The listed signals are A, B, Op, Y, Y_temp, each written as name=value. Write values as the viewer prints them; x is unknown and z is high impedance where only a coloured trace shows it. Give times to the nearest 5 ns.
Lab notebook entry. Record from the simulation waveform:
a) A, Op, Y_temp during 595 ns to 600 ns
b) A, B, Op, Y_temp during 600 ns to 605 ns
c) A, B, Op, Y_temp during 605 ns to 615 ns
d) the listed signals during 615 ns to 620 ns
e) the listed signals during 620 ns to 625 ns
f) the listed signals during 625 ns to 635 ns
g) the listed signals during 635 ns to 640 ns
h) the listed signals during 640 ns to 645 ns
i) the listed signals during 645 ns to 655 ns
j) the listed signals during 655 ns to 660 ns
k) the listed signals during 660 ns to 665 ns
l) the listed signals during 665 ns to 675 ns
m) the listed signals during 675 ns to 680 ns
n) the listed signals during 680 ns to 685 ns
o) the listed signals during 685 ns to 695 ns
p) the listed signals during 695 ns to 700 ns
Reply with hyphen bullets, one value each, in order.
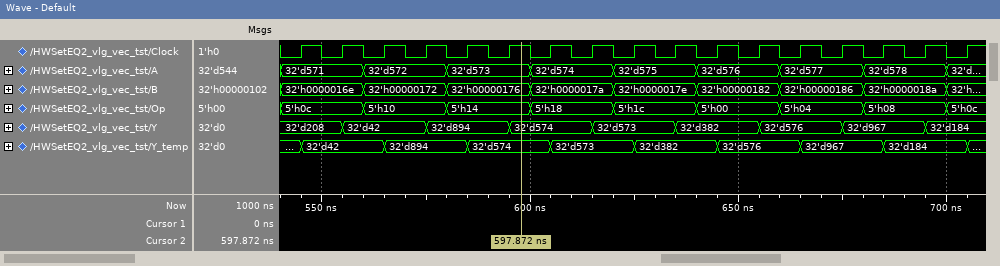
- A=32'd573, Op=5'h14, Y_temp=32'd574
- A=32'd574, B=32'h0000017a, Op=5'h18, Y_temp=32'd574
- A=32'd574, B=32'h0000017a, Op=5'h18, Y_temp=32'd573
- A=32'd574, B=32'h0000017a, Op=5'h18, Y=32'd573, Y_temp=32'd573
- A=32'd575, B=32'h0000017e, Op=5'h1c, Y=32'd573, Y_temp=32'd573
- A=32'd575, B=32'h0000017e, Op=5'h1c, Y=32'd573, Y_temp=32'd382
- A=32'd575, B=32'h0000017e, Op=5'h1c, Y=32'd382, Y_temp=32'd382
- A=32'd576, B=32'h00000182, Op=5'h00, Y=32'd382, Y_temp=32'd382
- A=32'd576, B=32'h00000182, Op=5'h00, Y=32'd382, Y_temp=32'd576
- A=32'd576, B=32'h00000182, Op=5'h00, Y=32'd576, Y_temp=32'd576
- A=32'd577, B=32'h00000186, Op=5'h04, Y=32'd576, Y_temp=32'd576
- A=32'd577, B=32'h00000186, Op=5'h04, Y=32'd576, Y_temp=32'd967
- A=32'd577, B=32'h00000186, Op=5'h04, Y=32'd967, Y_temp=32'd967
- A=32'd578, B=32'h0000018a, Op=5'h08, Y=32'd967, Y_temp=32'd967
- A=32'd578, B=32'h0000018a, Op=5'h08, Y=32'd967, Y_temp=32'd184
- A=32'd578, B=32'h0000018a, Op=5'h08, Y=32'd184, Y_temp=32'd184
